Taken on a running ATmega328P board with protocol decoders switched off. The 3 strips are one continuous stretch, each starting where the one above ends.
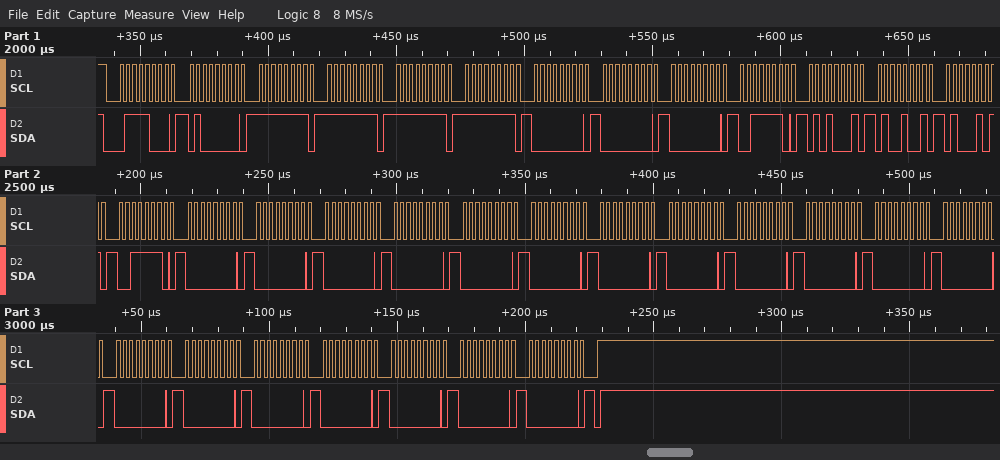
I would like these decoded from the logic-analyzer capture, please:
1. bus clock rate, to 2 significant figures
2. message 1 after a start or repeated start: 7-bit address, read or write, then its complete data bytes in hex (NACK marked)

400 kHz
0x3C write: 40 FF FF FF FF 00 00 00 3E 51 49 45 3E 00 00 00 00 00 00 00 00 00 00 00 00 00 00 00 00 00 00 00
